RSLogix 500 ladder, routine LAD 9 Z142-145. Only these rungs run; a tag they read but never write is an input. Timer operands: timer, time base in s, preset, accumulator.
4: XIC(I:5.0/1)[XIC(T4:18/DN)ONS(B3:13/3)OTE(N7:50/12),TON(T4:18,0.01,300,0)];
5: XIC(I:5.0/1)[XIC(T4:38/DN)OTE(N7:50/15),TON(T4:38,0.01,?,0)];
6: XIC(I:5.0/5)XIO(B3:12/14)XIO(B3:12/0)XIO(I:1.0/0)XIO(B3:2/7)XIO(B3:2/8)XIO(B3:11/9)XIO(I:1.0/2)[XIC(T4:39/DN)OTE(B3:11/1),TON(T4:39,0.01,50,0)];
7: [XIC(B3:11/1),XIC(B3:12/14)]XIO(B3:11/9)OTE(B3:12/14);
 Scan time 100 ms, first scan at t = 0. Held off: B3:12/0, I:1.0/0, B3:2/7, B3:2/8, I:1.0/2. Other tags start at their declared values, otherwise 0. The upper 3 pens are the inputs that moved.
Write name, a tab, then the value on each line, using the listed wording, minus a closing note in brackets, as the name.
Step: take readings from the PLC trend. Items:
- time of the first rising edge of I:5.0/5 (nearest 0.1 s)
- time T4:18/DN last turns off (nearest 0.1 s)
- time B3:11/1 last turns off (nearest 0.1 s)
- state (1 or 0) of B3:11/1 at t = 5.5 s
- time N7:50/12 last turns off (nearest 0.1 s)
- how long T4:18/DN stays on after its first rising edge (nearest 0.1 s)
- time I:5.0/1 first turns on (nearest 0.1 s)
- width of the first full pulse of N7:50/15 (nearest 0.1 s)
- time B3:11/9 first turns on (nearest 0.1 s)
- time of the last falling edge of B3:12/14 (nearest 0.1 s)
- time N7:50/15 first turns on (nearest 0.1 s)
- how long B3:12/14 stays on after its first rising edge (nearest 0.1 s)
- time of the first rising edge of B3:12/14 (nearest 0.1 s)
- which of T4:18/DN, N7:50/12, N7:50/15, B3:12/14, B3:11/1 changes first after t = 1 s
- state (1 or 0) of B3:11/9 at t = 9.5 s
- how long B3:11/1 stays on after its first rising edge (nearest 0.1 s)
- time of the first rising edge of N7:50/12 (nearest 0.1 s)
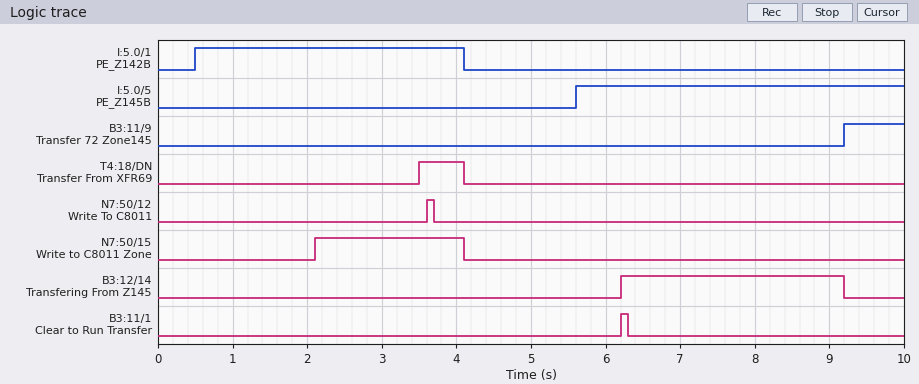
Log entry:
time of the first rising edge of I:5.0/5	5.6 s
time T4:18/DN last turns off	4.1 s
time B3:11/1 last turns off	6.3 s
state (1 or 0) of B3:11/1 at t = 5.5 s	0
time N7:50/12 last turns off	3.7 s
how long T4:18/DN stays on after its first rising edge	0.6 s
time I:5.0/1 first turns on	0.5 s
width of the first full pulse of N7:50/15	2.0 s
time B3:11/9 first turns on	9.2 s
time of the last falling edge of B3:12/14	9.2 s
time N7:50/15 first turns on	2.1 s
how long B3:12/14 stays on after its first rising edge	3.0 s
time of the first rising edge of B3:12/14	6.2 s
which of T4:18/DN, N7:50/12, N7:50/15, B3:12/14, B3:11/1 changes first after t = 1 s	N7:50/15
state (1 or 0) of B3:11/9 at t = 9.5 s	1
how long B3:11/1 stays on after its first rising edge	0.1 s
time of the first rising edge of N7:50/12	3.6 s
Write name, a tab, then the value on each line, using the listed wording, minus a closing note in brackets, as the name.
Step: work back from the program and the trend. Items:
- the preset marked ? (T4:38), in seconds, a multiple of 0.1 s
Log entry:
the preset marked ? (T4:38), in seconds, a multiple of 0.1 s	1.5 s
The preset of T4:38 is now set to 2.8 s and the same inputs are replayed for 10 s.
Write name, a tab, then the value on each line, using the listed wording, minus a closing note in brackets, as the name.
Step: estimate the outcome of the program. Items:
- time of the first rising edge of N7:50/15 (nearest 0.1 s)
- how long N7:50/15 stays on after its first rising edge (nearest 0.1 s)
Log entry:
time of the first rising edge of N7:50/15	3.4 s
how long N7:50/15 stays on after its first rising edge	0.7 s
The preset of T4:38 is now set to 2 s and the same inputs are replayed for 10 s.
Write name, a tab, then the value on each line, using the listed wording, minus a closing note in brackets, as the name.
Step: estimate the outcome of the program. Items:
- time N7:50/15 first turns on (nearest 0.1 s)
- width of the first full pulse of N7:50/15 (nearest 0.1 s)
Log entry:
time N7:50/15 first turns on	2.6 s
width of the first full pulse of N7:50/15	1.5 s
